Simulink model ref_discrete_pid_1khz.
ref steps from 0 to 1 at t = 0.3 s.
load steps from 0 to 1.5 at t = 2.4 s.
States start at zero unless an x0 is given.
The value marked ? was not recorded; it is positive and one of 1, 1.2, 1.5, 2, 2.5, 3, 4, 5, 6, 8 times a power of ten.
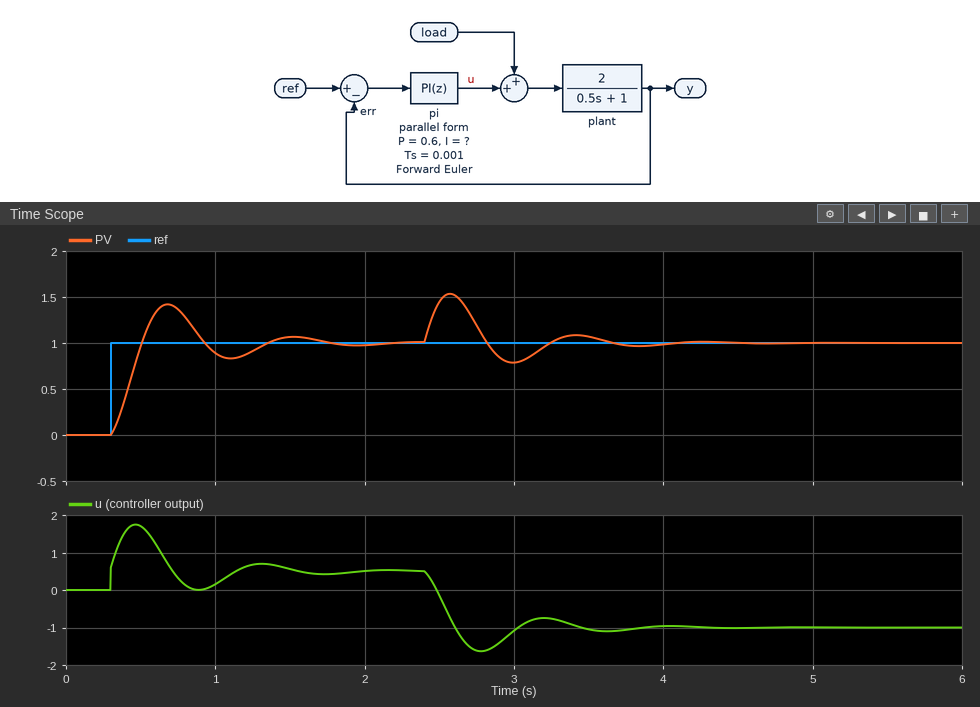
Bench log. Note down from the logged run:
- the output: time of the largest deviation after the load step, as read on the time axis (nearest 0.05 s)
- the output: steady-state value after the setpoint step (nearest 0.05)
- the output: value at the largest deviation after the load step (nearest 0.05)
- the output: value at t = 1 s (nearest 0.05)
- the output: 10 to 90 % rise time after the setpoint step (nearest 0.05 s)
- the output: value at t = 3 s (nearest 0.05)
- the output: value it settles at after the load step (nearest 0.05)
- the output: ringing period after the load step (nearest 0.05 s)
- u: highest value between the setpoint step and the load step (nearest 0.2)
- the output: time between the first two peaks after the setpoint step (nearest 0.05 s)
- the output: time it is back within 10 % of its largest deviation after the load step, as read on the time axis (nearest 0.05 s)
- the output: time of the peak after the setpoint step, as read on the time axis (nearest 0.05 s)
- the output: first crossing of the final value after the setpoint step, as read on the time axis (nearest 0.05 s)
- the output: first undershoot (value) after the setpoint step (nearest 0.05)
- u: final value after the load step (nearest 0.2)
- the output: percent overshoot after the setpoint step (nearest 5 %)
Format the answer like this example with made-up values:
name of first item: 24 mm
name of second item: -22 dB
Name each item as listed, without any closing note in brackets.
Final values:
the output: time of the largest deviation after the load step, as read on the time axis: 2.55 s
the output: steady-state value after the setpoint step: 1.00
the output: value at the largest deviation after the load step: 1.55
the output: value at t = 1 s: 0.90
the output: 10 to 90 % rise time after the setpoint step: 0.15 s
the output: value at t = 3 s: 0.80
the output: value it settles at after the load step: 1.00
the output: ringing period after the load step: 0.85 s
u: highest value between the setpoint step and the load step: 1.8
the output: time between the first two peaks after the setpoint step: 0.85 s
the output: time it is back within 10 % of its largest deviation after the load step, as read on the time axis: 3.55 s
the output: time of the peak after the setpoint step, as read on the time axis: 0.70 s
the output: first crossing of the final value after the setpoint step, as read on the time axis: 0.50 s
the output: first undershoot (value) after the setpoint step: 0.85
u: final value after the load step: -1.0
the output: percent overshoot after the setpoint step: 40 %
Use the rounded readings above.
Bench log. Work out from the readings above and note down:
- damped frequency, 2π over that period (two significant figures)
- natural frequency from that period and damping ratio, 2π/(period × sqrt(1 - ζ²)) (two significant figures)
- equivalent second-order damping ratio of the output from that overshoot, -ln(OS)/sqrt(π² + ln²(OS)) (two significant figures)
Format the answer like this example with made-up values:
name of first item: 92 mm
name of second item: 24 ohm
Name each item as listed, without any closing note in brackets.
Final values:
damped frequency, 2π over that period: 7.4 rad/s
natural frequency from that period and damping ratio, 2π/(period × sqrt(1 - ζ²)): 7.7 rad/s
equivalent second-order damping ratio of the output from that overshoot, -ln(OS)/sqrt(π² + ln²(OS)): 0.28
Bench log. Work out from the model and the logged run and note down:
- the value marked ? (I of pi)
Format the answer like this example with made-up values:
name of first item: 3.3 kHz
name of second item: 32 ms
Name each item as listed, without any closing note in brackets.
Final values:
the value marked ?: 15
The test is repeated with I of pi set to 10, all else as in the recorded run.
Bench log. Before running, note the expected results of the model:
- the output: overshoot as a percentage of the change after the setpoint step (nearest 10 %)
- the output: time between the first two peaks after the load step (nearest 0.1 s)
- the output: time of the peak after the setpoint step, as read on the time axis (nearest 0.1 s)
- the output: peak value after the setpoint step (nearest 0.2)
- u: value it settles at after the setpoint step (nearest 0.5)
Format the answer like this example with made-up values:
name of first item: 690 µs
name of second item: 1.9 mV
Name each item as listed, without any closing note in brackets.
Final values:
the output: overshoot as a percentage of the change after the setpoint step: 30 %
the output: time between the first two peaks after the load step: 1.1 s
the output: time of the peak after the setpoint step, as read on the time axis: 0.8 s
the output: peak value after the setpoint step: 1.4
u: value it settles at after the setpoint step: 0.5
